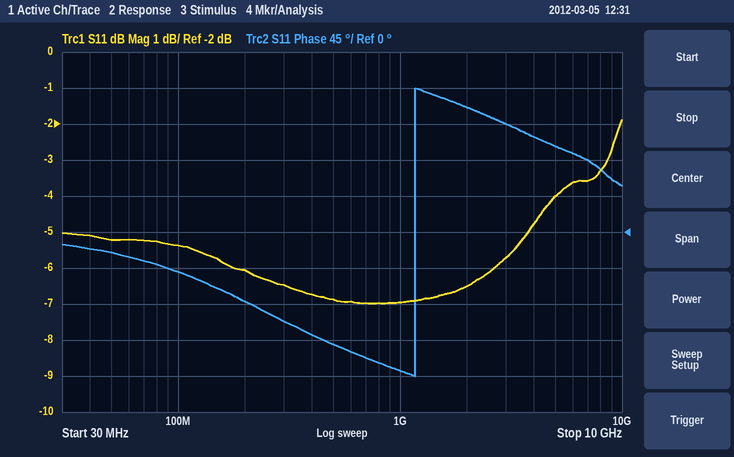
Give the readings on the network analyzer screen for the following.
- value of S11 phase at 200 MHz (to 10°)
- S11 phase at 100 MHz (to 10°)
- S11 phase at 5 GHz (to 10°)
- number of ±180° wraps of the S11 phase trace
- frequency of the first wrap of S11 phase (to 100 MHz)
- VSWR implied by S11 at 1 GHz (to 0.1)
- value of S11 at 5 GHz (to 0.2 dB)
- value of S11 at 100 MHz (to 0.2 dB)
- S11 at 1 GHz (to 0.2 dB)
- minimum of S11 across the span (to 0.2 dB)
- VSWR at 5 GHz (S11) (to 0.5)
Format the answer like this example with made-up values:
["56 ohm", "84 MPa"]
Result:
["-90°", "-50°", "110°", "1", "1.2 GHz", "2.6", "-4.0 dB", "-5.4 dB", "-7.0 dB", "-7.0 dB", "4.5"]
